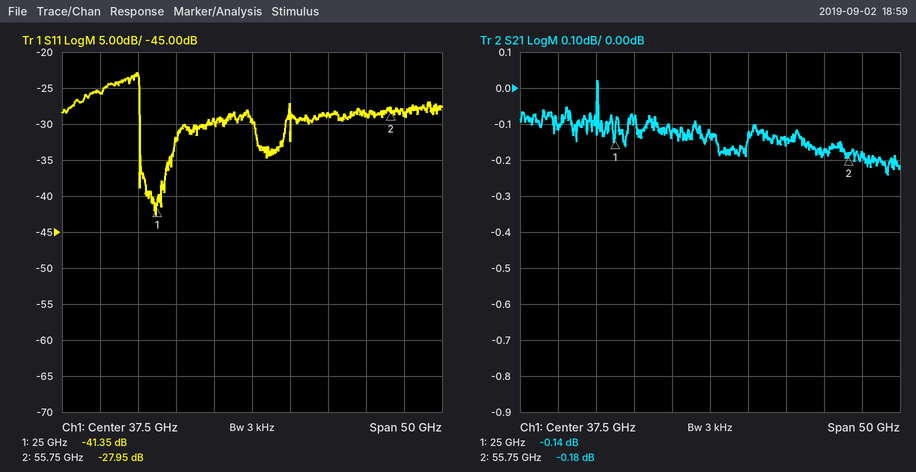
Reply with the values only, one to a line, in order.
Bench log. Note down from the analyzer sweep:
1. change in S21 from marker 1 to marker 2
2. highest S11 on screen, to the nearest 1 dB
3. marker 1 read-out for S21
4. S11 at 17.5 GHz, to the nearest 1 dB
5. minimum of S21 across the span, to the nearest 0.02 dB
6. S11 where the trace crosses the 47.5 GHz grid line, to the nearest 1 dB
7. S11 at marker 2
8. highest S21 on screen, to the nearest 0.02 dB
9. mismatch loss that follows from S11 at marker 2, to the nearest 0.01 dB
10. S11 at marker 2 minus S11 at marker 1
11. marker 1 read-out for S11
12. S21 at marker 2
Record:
-0.04 dB
-23 dB
-0.14 dB
-26 dB
-0.24 dB
-29 dB
-27.95 dB
0.02 dB
0.01 dB
13.40 dB
-41.35 dB
-0.18 dB
